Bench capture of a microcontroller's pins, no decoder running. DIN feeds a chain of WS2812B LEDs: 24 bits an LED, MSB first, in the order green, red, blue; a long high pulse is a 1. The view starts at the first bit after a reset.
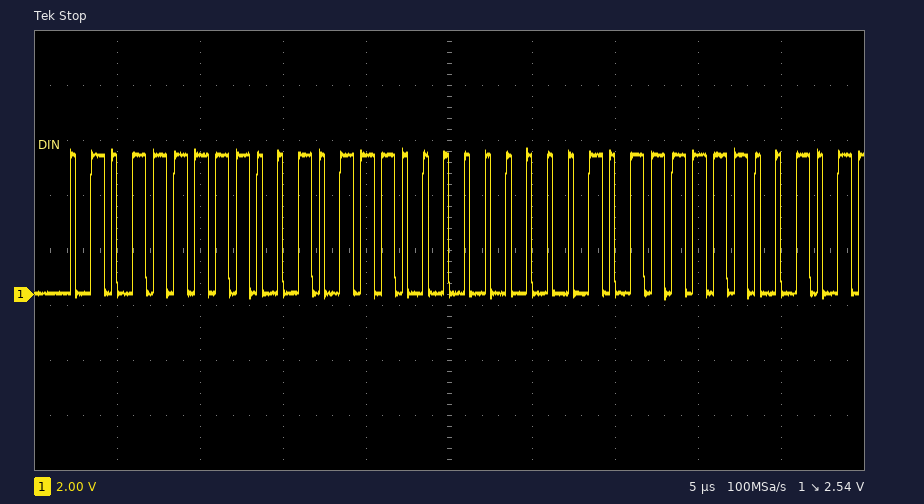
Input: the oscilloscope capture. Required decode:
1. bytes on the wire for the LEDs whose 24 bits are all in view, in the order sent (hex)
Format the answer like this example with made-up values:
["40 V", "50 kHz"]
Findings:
["5F 97 00"]
